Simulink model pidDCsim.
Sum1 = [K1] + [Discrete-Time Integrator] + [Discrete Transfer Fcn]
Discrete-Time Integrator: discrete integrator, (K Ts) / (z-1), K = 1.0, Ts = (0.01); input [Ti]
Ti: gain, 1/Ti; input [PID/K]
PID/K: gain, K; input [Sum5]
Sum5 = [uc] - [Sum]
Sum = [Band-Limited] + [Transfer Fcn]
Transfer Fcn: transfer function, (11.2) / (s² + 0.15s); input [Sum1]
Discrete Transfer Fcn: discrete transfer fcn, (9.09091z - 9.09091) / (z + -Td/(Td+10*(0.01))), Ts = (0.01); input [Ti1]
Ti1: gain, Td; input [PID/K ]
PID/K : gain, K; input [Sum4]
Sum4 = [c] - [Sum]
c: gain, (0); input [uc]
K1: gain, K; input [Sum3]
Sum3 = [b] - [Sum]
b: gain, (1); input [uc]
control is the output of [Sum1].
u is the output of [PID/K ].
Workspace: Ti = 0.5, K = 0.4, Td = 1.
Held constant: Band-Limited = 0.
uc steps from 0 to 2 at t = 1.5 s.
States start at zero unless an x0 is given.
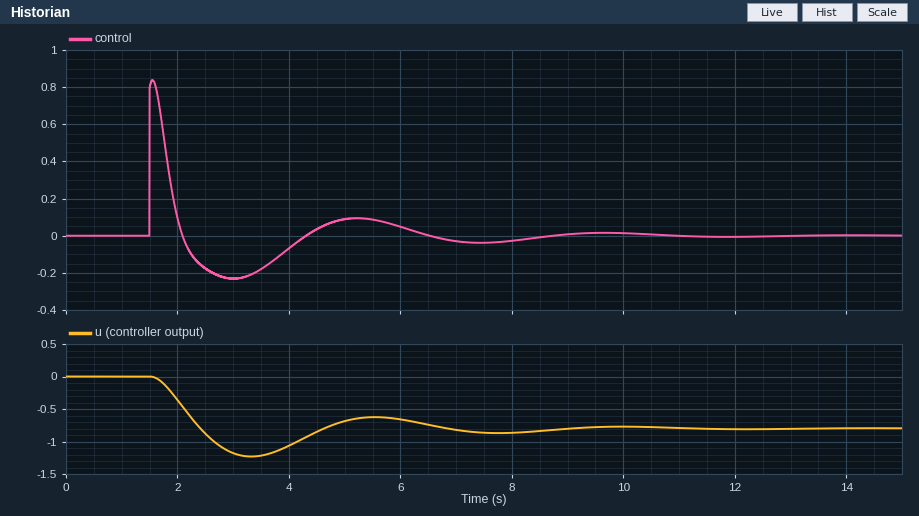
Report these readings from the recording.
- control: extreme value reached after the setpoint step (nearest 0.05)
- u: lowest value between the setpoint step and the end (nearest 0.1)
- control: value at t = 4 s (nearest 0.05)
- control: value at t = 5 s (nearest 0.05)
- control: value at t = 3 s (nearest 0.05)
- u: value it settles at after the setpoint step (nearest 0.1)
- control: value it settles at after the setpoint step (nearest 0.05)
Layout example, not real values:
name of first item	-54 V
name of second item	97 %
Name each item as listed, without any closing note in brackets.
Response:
control: extreme value reached after the setpoint step	0.85
u: lowest value between the setpoint step and the end	-1.2
control: value at t = 4 s	-0.05
control: value at t = 5 s	0.10
control: value at t = 3 s	-0.25
u: value it settles at after the setpoint step	-0.8
control: value it settles at after the setpoint step	0.00
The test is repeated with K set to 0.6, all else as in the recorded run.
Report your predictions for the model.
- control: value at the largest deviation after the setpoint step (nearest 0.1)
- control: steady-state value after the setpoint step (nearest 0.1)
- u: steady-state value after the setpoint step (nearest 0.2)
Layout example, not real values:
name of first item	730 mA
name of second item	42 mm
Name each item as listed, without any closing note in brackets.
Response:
control: value at the largest deviation after the setpoint step	1.2
control: steady-state value after the setpoint step	0.0
u: steady-state value after the setpoint step	-1.2
